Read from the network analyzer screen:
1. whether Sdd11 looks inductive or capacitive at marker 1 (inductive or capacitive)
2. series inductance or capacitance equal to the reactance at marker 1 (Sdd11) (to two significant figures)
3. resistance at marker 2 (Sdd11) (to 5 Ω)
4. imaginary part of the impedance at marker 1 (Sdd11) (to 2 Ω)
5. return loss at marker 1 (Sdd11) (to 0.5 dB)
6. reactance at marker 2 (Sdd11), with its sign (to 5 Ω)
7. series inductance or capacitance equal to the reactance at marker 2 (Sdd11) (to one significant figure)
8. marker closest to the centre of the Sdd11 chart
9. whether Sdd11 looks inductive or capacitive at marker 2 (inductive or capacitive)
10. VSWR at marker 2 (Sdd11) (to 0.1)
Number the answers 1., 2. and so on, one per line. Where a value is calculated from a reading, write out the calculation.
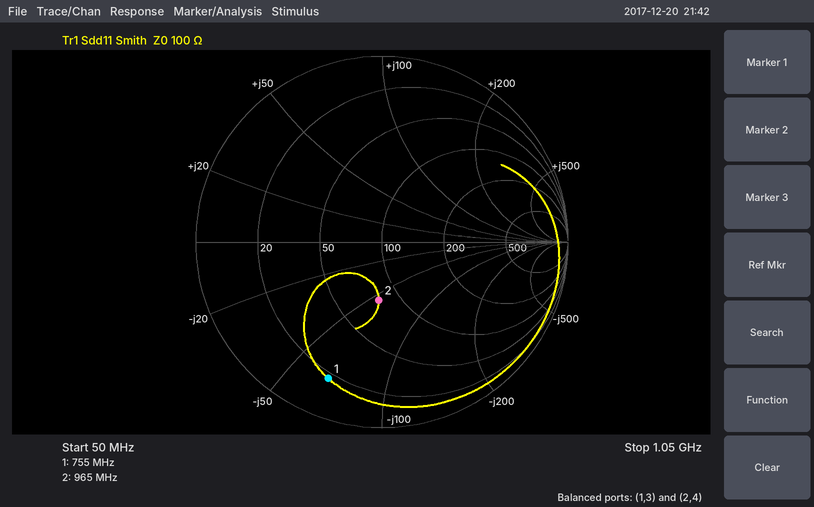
1. capacitive
2. C = 1/(2π × 755 MHz × 66 Ω) ≈ 3.2 pF
3. 80 Ω
4. -66 Ω
5. 2.0 dB
6. -55 Ω
7. C = 1/(2π × 965 MHz × 55 Ω) ≈ 3 pF
8. marker 2
9. capacitive
10. 1.9
